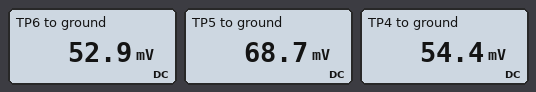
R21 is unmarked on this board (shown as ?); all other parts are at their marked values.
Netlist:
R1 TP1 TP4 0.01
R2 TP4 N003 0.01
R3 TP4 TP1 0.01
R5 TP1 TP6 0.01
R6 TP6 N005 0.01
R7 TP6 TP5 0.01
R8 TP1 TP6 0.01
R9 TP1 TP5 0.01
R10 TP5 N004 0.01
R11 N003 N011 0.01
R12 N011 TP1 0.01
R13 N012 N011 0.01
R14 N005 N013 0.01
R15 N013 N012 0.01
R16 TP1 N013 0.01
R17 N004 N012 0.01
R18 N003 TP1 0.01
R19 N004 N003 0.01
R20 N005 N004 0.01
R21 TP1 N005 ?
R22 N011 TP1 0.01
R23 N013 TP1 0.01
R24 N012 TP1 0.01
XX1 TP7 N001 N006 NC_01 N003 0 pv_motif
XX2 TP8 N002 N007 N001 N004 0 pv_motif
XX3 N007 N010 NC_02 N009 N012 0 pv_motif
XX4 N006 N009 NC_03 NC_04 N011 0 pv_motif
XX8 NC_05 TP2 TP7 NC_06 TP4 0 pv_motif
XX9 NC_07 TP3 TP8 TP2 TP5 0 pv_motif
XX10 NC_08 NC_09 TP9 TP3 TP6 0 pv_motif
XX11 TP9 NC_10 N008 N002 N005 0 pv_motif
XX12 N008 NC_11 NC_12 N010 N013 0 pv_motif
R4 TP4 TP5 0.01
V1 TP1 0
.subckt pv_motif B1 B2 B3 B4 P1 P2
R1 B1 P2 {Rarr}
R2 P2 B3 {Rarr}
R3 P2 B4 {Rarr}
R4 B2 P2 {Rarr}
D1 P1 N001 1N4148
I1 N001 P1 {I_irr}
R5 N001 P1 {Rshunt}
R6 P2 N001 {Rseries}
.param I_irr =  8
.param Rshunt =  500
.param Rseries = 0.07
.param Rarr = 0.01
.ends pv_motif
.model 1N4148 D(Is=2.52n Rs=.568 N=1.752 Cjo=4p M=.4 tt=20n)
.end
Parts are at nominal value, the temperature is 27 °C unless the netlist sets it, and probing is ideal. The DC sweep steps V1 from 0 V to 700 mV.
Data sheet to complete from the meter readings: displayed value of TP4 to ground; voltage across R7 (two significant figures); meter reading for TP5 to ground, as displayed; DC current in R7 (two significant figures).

54.4 mV
16 mV
68.7 mV
1.6 A
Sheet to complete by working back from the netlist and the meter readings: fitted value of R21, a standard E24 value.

7.5 mΩ
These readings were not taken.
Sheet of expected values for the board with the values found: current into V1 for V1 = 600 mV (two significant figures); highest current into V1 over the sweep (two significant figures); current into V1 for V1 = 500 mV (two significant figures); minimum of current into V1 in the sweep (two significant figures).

67 A
72 A
68 A
66 A
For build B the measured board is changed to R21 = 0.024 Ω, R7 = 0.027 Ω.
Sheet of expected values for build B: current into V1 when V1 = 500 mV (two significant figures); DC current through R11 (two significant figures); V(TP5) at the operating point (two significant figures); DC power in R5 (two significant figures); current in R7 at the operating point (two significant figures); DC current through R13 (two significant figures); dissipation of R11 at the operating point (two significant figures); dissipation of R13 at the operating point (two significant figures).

68 A
1.6 A
76 mV
330 mW
670 mA
1.7 A
26 mW
28 mW
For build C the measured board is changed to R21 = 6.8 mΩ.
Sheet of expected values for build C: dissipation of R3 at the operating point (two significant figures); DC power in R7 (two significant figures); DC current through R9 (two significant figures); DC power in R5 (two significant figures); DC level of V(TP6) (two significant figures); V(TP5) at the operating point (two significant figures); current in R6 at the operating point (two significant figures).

290 mW
26 mW
6.8 A
270 mW
52 mV
68 mV
840 mA
